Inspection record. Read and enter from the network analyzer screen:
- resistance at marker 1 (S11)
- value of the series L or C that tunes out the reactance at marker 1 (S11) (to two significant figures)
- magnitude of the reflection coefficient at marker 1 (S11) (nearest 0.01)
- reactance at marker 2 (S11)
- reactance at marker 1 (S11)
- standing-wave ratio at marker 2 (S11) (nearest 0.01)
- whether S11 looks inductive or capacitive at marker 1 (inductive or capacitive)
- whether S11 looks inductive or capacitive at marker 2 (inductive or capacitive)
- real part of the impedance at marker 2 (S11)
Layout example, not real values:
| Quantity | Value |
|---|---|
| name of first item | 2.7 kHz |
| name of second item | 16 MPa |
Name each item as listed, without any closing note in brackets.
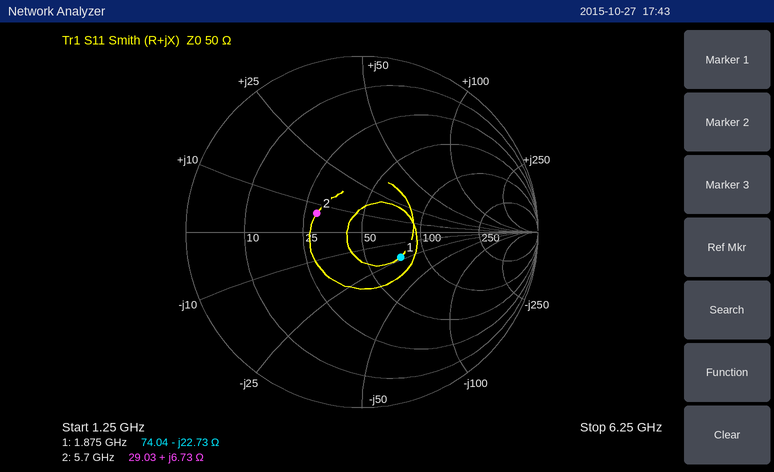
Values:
| Quantity | Value |
|---|---|
| resistance at marker 1 | 74.04 Ω |
| value of the series L or C that tunes out the reactance at marker 1 (S11) | 1.9 nH |
| magnitude of the reflection coefficient at marker 1 (S11) | 0.26 |
| reactance at marker 2 | +6.73 Ω |
| reactance at marker 1 | -22.73 Ω |
| standing-wave ratio at marker 2 (S11) | 1.77 |
| whether S11 looks inductive or capacitive at marker 1 | capacitive |
| whether S11 looks inductive or capacitive at marker 2 | inductive |
| real part of the impedance at marker 2 | 29.03 Ω |
